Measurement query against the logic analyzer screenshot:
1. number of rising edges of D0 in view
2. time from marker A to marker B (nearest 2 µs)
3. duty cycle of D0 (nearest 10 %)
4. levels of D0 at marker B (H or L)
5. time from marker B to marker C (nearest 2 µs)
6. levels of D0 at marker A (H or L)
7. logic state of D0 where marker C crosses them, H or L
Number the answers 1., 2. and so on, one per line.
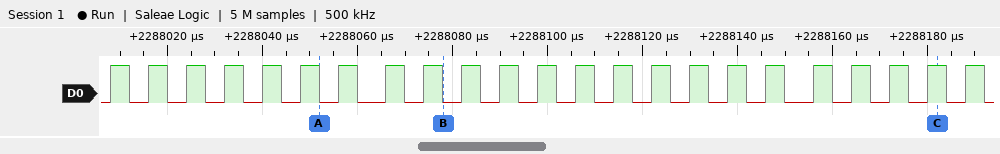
1. 23
2. 26 µs
3. 50 %
4. D0=L
5. 104 µs
6. D0=L
7. D0=H
